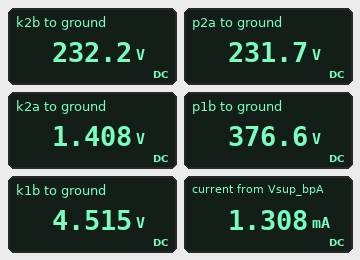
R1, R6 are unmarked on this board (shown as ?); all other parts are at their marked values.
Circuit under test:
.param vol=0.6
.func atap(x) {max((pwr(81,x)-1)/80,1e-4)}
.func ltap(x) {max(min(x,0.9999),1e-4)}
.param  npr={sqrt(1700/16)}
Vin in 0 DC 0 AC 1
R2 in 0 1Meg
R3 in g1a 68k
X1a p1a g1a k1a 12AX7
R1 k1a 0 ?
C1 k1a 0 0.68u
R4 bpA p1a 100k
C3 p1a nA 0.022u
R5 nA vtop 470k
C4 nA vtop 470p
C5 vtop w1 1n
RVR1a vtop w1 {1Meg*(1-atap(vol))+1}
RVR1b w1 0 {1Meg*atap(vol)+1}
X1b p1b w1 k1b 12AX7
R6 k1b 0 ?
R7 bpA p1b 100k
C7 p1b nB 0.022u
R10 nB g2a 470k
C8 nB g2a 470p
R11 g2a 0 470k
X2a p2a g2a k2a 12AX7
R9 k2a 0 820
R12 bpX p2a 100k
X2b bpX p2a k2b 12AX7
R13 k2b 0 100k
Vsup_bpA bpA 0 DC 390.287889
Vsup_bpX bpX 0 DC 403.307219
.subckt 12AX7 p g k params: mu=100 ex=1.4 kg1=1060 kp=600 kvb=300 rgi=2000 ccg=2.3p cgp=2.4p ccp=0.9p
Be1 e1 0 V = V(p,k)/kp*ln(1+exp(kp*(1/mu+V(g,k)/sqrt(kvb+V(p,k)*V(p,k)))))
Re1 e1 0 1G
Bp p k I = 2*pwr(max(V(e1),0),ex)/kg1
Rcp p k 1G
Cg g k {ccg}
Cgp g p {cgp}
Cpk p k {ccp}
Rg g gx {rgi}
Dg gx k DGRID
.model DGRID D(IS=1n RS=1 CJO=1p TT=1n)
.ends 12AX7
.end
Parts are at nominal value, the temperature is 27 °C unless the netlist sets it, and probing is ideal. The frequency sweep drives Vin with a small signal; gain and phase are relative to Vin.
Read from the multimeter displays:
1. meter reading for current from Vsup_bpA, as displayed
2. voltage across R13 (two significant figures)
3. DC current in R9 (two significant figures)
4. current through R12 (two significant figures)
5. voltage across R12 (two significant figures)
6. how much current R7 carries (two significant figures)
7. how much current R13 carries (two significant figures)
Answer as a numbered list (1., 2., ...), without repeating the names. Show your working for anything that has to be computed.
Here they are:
1. 1.308 mA
2. 232.2 V = 230 V
3. (1.408 V) / 820 Ω = 1.7 mA
4. (403.3 V - 231.7 V) / 100 kΩ = 1.7 mA
5. 403.3 V - 231.7 V = 170 V
6. (390.3 V - 376.6 V) / 100 kΩ = 140 µA
7. (232.2 V) / 100 kΩ = 2.3 mA
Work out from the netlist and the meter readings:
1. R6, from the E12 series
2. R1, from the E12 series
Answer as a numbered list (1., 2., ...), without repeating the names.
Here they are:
1. 33 kΩ
2. 1.8 kΩ
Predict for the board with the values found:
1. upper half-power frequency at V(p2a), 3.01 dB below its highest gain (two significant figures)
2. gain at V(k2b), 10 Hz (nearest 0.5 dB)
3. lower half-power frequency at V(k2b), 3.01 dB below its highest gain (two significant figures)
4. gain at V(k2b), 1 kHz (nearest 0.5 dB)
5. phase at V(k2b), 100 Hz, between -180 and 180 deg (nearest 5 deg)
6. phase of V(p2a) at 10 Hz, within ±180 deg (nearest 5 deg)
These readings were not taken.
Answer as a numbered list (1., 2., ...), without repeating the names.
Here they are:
1. 16 kHz
2. 41.0 dB
3. 2.3 kHz
4. 61.0 dB
5. -135 deg
6. -115 deg
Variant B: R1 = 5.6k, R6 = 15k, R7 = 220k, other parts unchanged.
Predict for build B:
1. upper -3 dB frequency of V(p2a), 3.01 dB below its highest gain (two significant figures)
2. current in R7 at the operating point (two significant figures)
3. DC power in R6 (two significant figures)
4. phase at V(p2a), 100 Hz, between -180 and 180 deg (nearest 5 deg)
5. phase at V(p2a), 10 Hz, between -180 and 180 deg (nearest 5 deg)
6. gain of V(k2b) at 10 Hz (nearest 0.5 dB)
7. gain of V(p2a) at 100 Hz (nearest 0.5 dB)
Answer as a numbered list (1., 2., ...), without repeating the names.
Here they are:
1. 14 kHz
2. 250 µA
3. 910 µW
4. -120 deg
5. -110 deg
6. 46.0 dB
7. 55.5 dB
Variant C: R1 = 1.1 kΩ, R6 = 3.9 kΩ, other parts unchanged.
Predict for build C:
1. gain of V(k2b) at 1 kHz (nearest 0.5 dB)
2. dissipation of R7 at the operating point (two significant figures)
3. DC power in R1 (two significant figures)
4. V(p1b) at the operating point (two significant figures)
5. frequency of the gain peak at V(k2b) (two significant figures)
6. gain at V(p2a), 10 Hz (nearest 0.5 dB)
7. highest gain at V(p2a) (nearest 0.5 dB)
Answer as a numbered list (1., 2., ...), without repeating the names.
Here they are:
1. 78.0 dB
2. 54 mW
3. 2.4 mW
4. 320 V
5. 6.0 kHz
6. 60.0 dB
7. 86.5 dB
